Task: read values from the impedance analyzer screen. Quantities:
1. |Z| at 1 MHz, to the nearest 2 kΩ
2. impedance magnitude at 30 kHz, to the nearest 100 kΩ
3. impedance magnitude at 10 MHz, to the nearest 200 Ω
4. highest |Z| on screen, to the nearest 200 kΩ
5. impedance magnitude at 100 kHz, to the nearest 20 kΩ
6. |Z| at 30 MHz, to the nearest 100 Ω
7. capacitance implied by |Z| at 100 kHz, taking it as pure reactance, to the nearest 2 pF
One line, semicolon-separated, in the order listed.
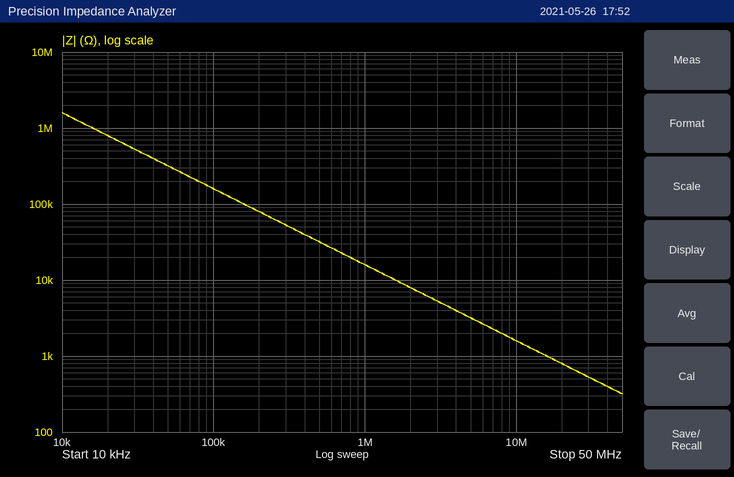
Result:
16 kΩ; 500 kΩ; 1.6 kΩ; 1.6 MΩ; 160 kΩ; 500 Ω; 10 pF
